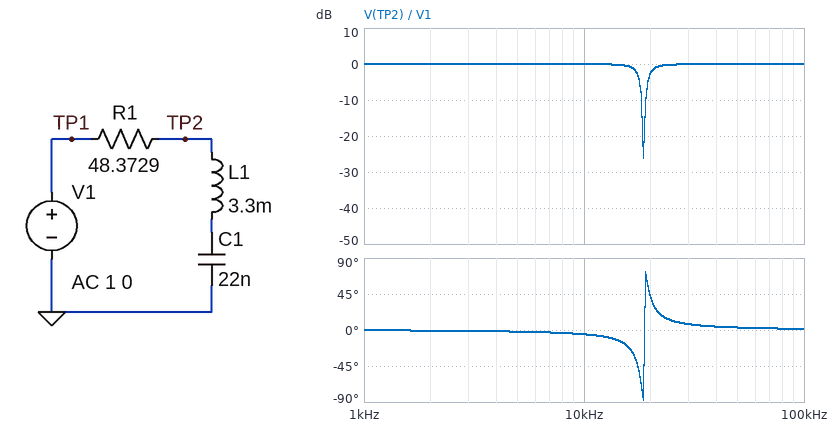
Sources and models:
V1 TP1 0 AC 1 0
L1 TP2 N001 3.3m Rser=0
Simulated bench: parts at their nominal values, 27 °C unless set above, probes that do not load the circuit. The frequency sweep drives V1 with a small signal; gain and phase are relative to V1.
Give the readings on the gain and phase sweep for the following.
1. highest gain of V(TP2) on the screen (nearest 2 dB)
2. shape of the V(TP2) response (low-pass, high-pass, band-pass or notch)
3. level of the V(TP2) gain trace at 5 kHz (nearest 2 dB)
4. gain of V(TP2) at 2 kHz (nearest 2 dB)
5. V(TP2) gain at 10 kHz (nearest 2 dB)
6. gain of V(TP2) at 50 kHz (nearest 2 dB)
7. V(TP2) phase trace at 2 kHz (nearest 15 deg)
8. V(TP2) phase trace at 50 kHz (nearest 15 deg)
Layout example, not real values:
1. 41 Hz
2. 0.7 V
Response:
1. 0 dB
2. notch
3. 0 dB
4. 0 dB
5. 0 dB
6. 0 dB
7. 0 deg
8. 0 deg
